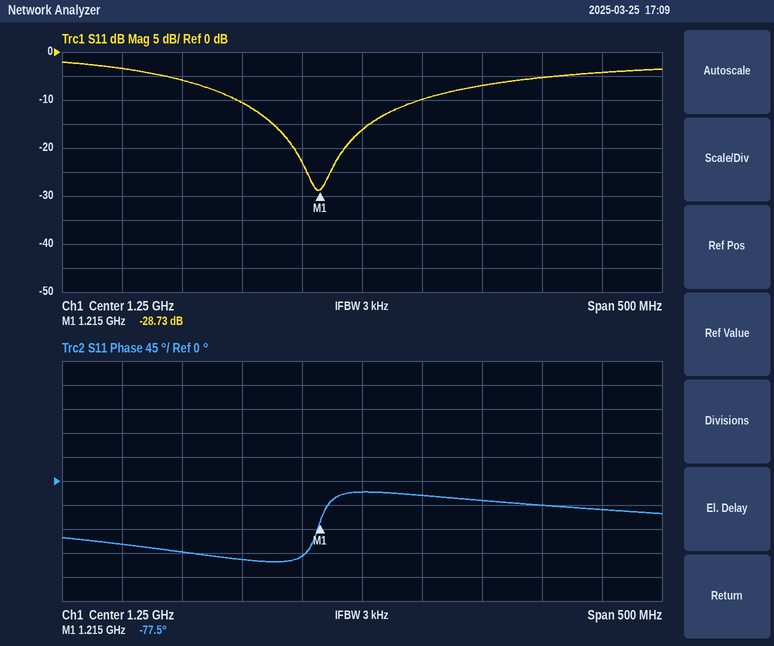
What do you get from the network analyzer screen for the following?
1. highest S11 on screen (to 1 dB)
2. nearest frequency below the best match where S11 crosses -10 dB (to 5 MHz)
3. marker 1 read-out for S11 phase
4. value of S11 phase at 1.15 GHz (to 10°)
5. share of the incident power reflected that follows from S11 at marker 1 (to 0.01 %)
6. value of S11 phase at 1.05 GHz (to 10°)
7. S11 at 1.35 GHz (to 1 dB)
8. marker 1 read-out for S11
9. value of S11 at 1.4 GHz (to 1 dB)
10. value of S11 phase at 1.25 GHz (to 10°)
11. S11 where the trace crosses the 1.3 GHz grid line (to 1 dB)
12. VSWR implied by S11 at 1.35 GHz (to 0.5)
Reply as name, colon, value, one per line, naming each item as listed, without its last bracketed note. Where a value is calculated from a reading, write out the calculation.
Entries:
highest S11 on screen: -2 dB
nearest frequency below the best match where S11 crosses -10 dB: 1.145 GHz
marker 1 read-out for S11 phase: -77.5°
value of S11 phase at 1.15 GHz: -150°
share of the incident power reflected that follows from S11 at marker 1: 10^(-28.73/10) ≈ 0.13 %
value of S11 phase at 1.05 GHz: -120°
S11 at 1.35 GHz: -7 dB
marker 1 read-out for S11: -28.73 dB
value of S11 at 1.4 GHz: -5 dB
value of S11 phase at 1.25 GHz: -20°
S11 where the trace crosses the 1.3 GHz grid line: -10 dB
VSWR implied by S11 at 1.35 GHz: |Γ| = 10^(-7/20) = 0.4467; VSWR = (1 + 0.4467)/(1 − 0.4467) ≈ 2.61, so 2.5 to the nearest 0.5
